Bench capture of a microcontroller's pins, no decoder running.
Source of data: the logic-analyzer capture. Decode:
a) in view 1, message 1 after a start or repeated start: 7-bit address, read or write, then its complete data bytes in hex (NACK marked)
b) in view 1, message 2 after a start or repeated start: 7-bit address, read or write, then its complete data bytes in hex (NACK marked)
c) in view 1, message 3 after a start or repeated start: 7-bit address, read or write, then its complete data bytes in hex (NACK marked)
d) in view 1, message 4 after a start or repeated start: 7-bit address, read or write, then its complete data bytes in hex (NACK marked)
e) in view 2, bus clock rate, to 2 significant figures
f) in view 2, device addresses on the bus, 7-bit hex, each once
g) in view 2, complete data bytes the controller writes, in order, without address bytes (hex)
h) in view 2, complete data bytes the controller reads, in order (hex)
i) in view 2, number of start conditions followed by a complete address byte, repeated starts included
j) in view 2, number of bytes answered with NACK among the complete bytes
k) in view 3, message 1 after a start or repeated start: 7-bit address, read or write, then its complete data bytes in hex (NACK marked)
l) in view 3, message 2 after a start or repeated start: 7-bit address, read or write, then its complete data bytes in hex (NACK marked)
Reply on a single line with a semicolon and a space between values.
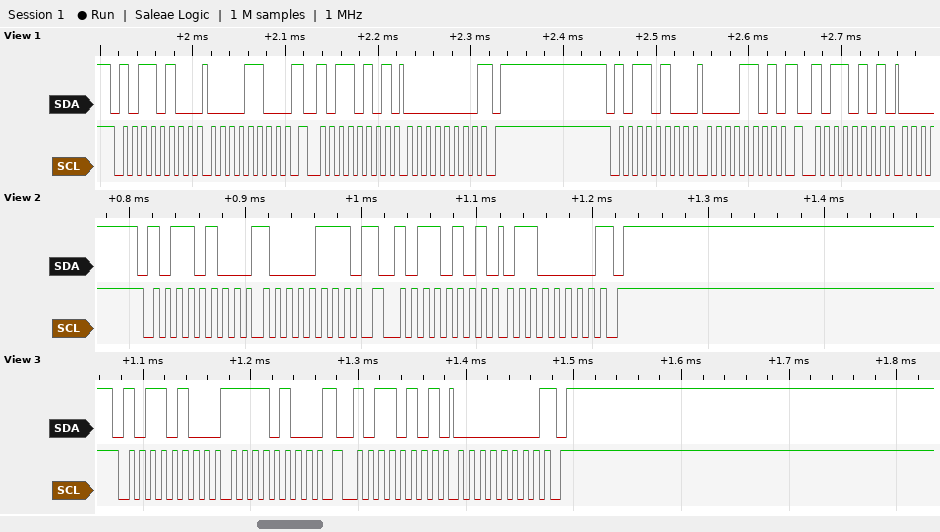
0x5A write: 0C; 0x5A read: 00 NACK; 0x5A write: 0D; 0x5A read; 100 kHz; 0x5A; 87; 60; 2; 1; 0x5A write: F4; 0x5A read: 00 NACK
